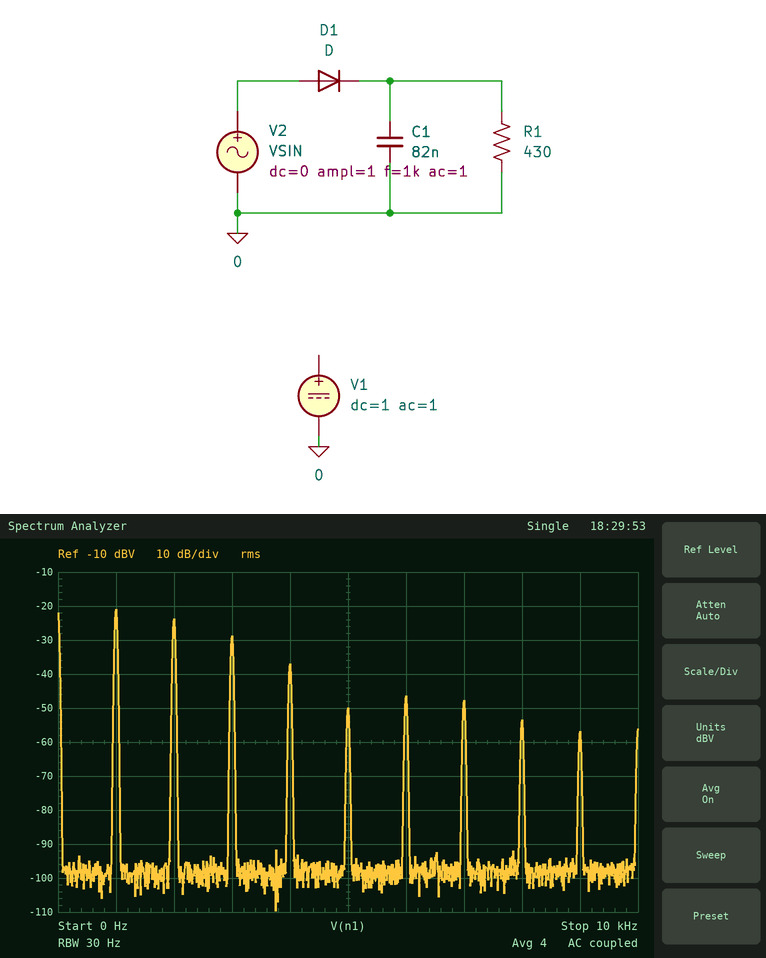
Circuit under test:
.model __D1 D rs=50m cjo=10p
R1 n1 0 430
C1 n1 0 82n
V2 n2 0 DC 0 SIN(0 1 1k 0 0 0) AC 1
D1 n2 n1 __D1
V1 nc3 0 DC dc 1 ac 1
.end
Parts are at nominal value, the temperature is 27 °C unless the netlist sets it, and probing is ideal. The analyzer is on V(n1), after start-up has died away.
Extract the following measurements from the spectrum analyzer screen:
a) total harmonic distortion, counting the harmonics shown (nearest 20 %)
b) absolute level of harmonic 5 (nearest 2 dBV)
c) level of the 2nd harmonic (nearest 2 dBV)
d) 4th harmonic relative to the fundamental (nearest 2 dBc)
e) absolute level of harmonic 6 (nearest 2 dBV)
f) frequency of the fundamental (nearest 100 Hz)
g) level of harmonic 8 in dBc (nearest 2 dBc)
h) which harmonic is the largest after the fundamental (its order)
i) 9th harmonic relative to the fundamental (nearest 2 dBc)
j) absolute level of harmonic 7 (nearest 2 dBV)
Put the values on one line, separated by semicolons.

80 %; -50 dBV; -24 dBV; -16 dBc; -46 dBV; 1.0 kHz; -32 dBc; 2; -36 dBc; -48 dBV
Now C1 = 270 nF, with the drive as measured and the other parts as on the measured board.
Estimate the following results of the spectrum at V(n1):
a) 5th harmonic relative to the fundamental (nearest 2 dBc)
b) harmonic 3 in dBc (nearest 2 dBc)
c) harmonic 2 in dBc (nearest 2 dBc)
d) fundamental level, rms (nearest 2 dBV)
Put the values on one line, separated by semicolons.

-24 dBc; -10 dBc; -4 dBc; -20 dBV
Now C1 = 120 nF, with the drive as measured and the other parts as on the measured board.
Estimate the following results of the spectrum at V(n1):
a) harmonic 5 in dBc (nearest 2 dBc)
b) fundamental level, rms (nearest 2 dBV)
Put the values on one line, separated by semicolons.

-26 dBc; -20 dBV
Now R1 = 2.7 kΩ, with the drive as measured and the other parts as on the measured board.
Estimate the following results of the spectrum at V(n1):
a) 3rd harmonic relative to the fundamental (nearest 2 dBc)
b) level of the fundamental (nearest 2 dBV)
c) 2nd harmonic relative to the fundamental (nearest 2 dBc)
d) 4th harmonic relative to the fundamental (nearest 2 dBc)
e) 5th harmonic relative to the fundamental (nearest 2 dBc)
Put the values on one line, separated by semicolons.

-12 dBc; -20 dBV; -6 dBc; -18 dBc; -24 dBc
